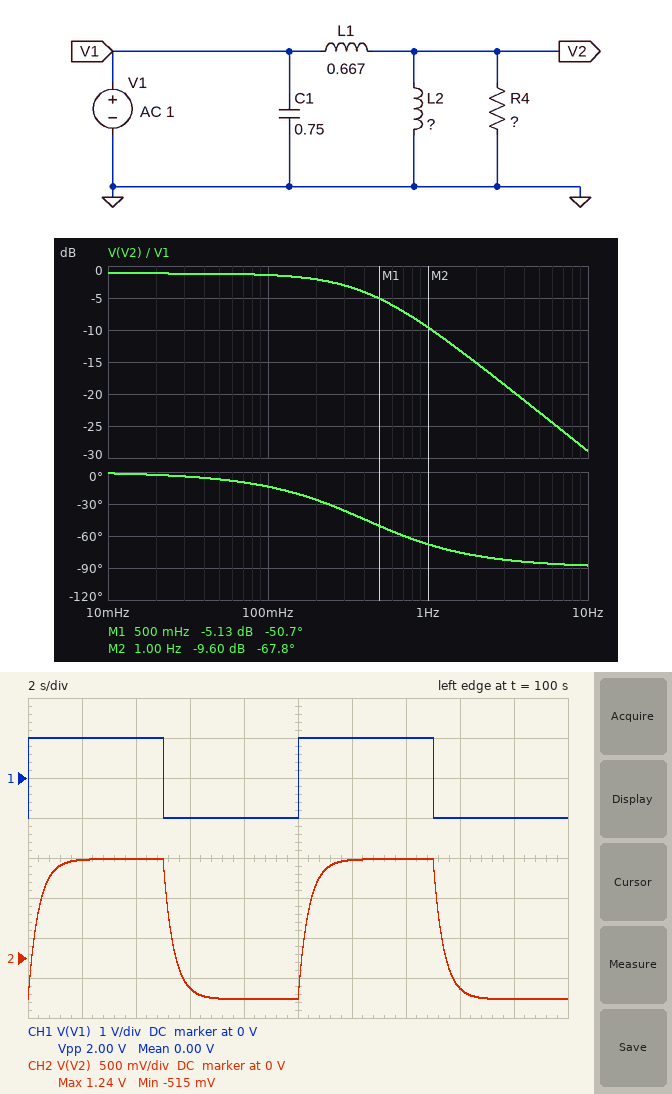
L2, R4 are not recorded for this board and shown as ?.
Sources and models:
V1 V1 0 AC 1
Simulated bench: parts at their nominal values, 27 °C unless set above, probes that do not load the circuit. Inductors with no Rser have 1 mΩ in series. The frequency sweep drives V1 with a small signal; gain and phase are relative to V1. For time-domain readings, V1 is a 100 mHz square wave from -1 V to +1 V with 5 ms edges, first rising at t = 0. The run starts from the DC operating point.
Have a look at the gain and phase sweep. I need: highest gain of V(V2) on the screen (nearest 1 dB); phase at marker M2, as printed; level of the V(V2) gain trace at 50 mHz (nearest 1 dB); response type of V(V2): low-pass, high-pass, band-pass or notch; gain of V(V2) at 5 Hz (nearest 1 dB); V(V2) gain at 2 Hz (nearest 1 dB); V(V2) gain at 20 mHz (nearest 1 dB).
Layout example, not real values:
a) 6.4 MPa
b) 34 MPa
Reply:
a) -1 dB
b) -67.8 deg
c) -1 dB
d) low-pass
e) -23 dB
f) -15 dB
g) -1 dB
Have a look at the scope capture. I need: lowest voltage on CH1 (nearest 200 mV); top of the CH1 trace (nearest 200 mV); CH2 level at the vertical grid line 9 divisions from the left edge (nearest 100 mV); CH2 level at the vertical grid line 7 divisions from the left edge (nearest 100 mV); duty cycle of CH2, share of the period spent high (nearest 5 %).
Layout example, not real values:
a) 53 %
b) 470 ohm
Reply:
a) -1.0 V
b) 1.0 V
c) -500 mV
d) 1.2 V
e) 50 %
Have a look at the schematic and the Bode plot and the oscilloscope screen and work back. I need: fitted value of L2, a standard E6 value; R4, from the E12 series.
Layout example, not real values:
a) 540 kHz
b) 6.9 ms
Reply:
a) 4.7 H
b) 1.5 Ω
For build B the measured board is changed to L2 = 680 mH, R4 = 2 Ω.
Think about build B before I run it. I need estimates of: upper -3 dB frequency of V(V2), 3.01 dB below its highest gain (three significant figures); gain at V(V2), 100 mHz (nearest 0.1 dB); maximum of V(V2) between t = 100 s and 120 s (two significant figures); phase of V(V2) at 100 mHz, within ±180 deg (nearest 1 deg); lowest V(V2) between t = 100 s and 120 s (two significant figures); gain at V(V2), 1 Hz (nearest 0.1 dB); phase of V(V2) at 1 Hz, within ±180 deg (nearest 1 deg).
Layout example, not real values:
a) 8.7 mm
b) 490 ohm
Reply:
a) 946 mHz
b) -6.0 dB
c) 510 mV
d) -6 deg
e) -500 mV
f) -9.2 dB
g) -47 deg
